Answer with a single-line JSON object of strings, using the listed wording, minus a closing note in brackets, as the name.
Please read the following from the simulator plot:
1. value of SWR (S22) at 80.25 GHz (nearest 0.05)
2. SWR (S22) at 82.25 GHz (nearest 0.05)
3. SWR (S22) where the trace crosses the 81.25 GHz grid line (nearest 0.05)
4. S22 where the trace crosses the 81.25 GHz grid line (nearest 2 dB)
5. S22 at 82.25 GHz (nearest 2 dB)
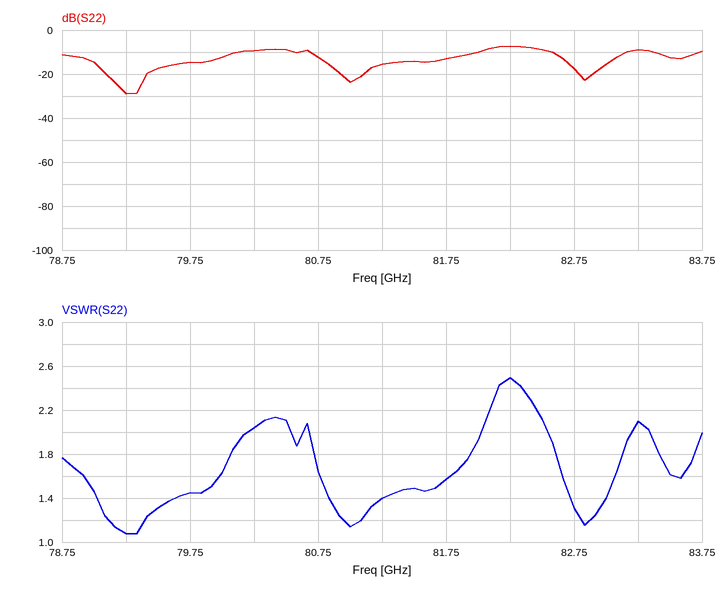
{"value of SWR (S22) at 80.25 GHz": "2.05", "SWR (S22) at 82.25 GHz": "2.50", "SWR (S22) where the trace crosses the 81.25 GHz grid line": "1.40", "S22 where the trace crosses the 81.25 GHz grid line": "-16 dB", "S22 at 82.25 GHz": "-8 dB"}
